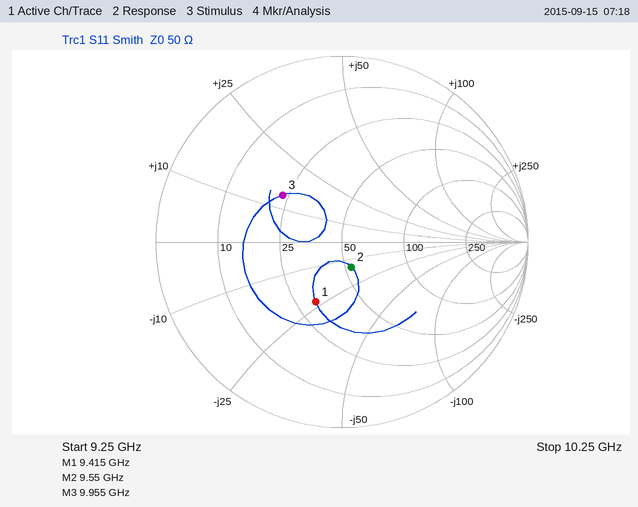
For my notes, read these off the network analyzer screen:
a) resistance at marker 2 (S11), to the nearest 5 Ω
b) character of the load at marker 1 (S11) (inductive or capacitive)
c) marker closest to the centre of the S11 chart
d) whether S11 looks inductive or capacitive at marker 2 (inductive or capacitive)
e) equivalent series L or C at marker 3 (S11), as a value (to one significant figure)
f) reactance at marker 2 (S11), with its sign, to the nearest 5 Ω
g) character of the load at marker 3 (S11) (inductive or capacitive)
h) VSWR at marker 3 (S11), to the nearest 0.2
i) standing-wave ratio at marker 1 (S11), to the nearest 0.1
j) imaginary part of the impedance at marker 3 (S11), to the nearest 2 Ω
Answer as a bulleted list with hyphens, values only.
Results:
- 55 Ω
- capacitive
- marker 2
- capacitive
- 200 pH
- -15 Ω
- inductive
- 2.4
- 2.1
- +14 Ω
